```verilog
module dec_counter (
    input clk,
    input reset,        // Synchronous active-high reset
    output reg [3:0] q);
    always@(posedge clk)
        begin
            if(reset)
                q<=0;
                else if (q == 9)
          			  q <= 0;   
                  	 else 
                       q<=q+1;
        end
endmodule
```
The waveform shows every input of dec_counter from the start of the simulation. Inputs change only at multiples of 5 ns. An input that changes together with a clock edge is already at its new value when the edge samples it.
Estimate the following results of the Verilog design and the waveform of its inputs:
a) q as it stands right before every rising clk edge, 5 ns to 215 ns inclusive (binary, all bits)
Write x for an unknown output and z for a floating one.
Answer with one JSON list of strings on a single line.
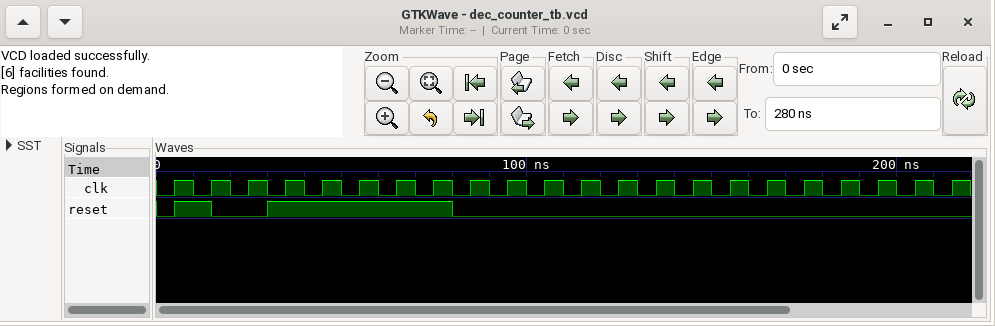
["x, 0000, 0001, 0010, 0000, 0000, 0000, 0000, 0000, 0001, 0010, 0011, 0100, 0101, 0110, 0111, 1000, 1001, 0000, 0001, 0010, 0011"]
